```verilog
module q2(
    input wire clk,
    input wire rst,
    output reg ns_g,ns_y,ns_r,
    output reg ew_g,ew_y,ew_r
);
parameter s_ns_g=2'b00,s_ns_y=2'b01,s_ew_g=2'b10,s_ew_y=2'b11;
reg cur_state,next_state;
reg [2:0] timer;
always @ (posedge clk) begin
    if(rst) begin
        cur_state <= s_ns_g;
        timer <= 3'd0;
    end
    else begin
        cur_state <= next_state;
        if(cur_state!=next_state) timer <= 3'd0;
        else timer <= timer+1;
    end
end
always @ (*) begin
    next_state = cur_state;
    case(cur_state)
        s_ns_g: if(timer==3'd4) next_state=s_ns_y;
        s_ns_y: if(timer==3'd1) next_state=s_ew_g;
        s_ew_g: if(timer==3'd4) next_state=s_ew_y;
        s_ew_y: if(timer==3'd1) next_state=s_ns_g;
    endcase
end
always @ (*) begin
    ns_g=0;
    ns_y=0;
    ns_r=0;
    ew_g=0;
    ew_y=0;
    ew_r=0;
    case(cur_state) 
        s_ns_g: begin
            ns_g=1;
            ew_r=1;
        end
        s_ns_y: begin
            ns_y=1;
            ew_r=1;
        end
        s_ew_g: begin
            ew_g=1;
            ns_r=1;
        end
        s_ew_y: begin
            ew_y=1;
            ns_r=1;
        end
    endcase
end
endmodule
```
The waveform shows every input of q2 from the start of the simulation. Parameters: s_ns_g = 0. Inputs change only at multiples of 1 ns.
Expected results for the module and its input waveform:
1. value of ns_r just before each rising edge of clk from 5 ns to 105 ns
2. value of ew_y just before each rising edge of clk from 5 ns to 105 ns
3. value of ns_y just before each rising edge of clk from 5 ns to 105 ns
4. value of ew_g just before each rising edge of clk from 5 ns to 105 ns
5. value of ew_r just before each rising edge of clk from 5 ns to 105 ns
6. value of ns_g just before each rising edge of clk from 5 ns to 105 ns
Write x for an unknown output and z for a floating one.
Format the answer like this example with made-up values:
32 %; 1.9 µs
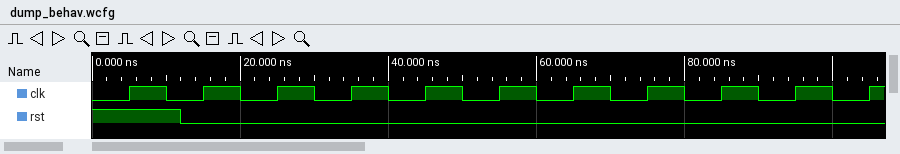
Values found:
x 0 0 0 0 0 0 0 0 0 0; x 0 0 0 0 0 0 0 0 0 0; x 0 0 0 0 0 1 1 0 0 0; x 0 0 0 0 0 0 0 0 0 0; x 1 1 1 1 1 1 1 1 1 1; x 1 1 1 1 1 0 0 1 1 1
